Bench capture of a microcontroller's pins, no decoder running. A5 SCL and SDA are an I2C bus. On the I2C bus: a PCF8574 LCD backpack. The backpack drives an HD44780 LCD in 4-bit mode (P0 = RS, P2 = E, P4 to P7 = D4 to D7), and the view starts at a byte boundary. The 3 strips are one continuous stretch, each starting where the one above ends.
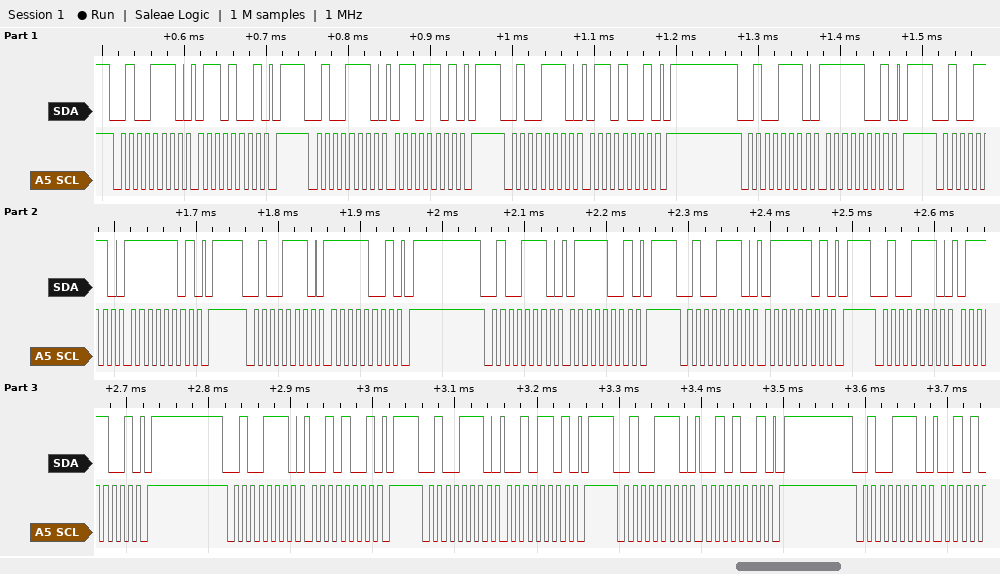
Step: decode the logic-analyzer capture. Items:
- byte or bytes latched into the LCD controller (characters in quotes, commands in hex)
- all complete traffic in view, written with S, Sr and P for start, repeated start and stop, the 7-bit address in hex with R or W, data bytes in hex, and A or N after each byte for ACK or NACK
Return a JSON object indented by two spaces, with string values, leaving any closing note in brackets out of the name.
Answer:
{
  "byte or bytes latched into the LCD controller": "'o' 'r'",
  "all complete traffic in view, written with S, Sr and P for start, repeated start and stop, the 7-bit address in hex with R or W, data bytes in hex, and A or N after each byte for ACK or NACK": "S 27W A 69 A P S 27W A 6D A P S 27W A 69 A P S 27W A F9 A P S 27W A FD A P S 27W A F9 A P S 27W A 79 A P S 27W A 7D A P S 27W A 79 A P S 27W A 29 A P S 27W A 2D A P S 27W A 29 A P S 27W A"
}
